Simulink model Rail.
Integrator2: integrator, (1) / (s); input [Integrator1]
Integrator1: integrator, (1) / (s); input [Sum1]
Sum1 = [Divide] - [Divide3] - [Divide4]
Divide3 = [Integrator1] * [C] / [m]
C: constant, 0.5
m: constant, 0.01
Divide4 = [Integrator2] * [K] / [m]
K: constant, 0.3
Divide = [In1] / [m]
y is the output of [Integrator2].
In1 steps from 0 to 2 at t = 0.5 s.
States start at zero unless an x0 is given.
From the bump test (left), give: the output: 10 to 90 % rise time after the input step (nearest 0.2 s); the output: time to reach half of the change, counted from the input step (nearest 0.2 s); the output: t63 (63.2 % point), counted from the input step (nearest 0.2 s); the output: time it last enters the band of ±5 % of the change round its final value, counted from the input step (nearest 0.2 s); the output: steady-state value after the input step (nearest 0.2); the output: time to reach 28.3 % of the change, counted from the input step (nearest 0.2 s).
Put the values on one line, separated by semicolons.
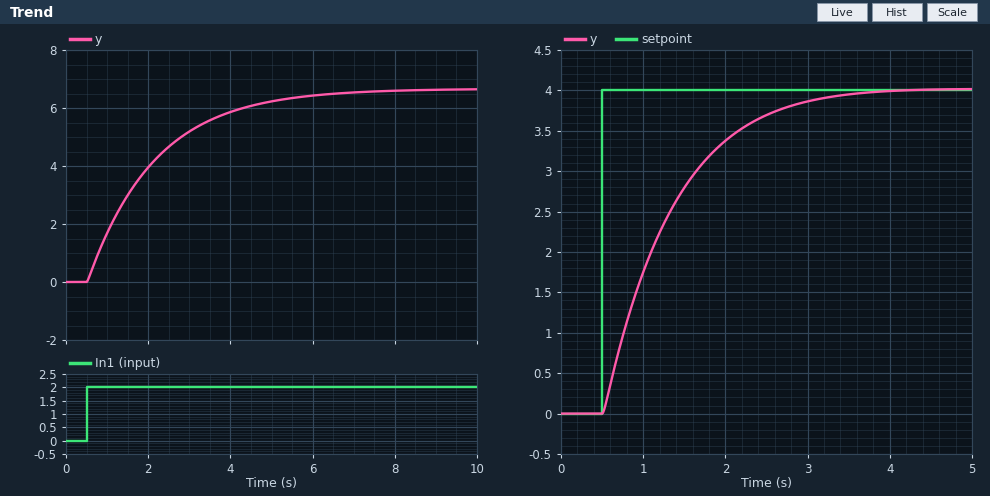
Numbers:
3.6 s; 1.2 s; 1.6 s; 5.0 s; 6.6; 0.6 s
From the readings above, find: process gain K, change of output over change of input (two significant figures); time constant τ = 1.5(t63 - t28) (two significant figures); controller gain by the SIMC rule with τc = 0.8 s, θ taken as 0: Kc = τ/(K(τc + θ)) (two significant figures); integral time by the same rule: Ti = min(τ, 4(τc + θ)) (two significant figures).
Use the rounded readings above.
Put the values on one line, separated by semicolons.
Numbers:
3.3; 1.5 s; 0.57; 1.5 s
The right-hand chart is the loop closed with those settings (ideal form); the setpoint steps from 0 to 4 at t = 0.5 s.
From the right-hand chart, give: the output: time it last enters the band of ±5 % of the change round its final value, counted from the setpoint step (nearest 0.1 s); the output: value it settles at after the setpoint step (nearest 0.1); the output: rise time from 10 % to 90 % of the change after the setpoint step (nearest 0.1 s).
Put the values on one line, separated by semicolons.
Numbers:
2.3 s; 4.0; 1.7 s
